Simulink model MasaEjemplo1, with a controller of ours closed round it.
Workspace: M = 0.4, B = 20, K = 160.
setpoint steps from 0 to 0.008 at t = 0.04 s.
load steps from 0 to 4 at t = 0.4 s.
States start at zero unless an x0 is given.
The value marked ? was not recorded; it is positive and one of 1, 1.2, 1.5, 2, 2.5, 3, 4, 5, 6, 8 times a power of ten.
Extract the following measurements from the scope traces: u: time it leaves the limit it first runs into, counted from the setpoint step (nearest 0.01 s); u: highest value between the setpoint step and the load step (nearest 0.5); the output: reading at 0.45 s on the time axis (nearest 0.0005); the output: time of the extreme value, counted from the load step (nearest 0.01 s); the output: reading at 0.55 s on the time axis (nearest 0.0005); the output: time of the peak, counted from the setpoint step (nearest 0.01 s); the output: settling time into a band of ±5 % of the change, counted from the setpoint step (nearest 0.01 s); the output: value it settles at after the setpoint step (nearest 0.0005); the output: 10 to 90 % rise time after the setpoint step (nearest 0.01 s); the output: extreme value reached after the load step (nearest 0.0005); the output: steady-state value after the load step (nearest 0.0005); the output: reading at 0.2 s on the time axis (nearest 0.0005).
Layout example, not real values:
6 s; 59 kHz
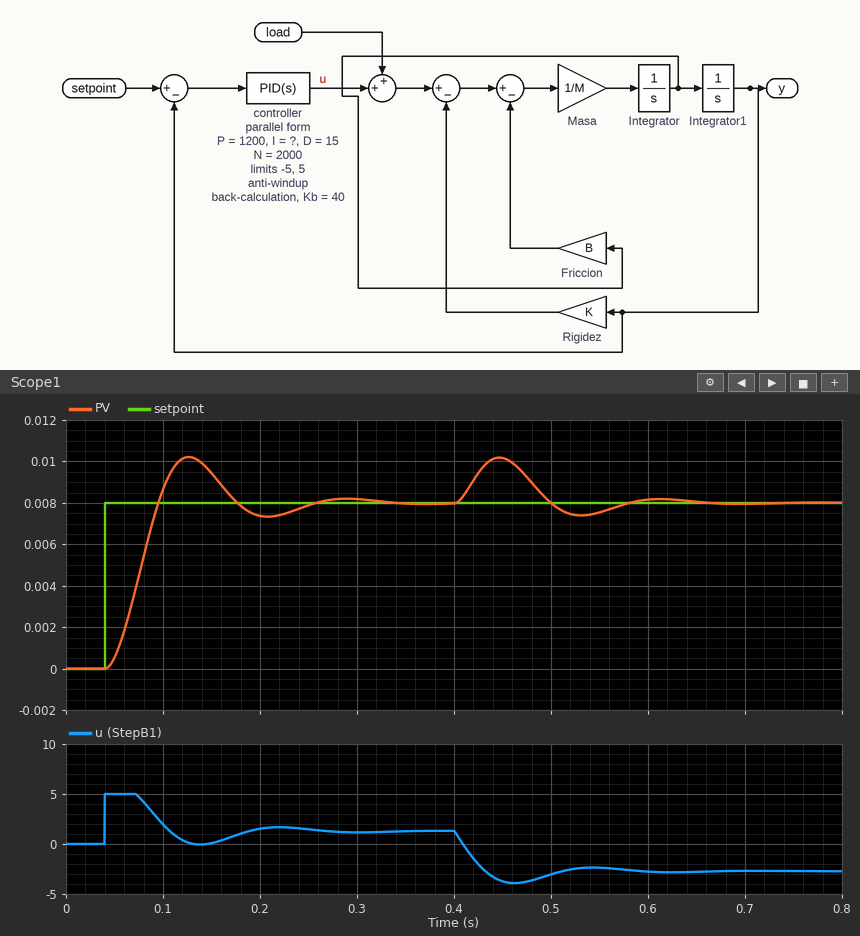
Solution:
0.03 s; 5.0; 0.0100; 0.05 s; 0.0075; 0.09 s; 0.19 s; 0.0080; 0.04 s; 0.0100; 0.0080; 0.0075
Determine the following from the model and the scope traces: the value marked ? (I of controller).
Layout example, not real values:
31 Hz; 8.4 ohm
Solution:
40000
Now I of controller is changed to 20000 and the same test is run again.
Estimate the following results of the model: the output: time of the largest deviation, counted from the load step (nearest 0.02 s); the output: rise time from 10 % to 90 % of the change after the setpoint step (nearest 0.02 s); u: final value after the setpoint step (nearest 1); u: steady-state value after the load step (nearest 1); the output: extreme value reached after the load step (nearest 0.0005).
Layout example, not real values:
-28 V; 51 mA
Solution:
0.06 s; 0.06 s; 1; -3; 0.0105
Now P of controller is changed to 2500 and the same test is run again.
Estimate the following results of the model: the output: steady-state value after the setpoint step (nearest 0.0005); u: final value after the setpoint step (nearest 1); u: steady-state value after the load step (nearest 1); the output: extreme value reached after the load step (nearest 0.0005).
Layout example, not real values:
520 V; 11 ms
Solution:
0.0080; 1; -3; 0.0095
